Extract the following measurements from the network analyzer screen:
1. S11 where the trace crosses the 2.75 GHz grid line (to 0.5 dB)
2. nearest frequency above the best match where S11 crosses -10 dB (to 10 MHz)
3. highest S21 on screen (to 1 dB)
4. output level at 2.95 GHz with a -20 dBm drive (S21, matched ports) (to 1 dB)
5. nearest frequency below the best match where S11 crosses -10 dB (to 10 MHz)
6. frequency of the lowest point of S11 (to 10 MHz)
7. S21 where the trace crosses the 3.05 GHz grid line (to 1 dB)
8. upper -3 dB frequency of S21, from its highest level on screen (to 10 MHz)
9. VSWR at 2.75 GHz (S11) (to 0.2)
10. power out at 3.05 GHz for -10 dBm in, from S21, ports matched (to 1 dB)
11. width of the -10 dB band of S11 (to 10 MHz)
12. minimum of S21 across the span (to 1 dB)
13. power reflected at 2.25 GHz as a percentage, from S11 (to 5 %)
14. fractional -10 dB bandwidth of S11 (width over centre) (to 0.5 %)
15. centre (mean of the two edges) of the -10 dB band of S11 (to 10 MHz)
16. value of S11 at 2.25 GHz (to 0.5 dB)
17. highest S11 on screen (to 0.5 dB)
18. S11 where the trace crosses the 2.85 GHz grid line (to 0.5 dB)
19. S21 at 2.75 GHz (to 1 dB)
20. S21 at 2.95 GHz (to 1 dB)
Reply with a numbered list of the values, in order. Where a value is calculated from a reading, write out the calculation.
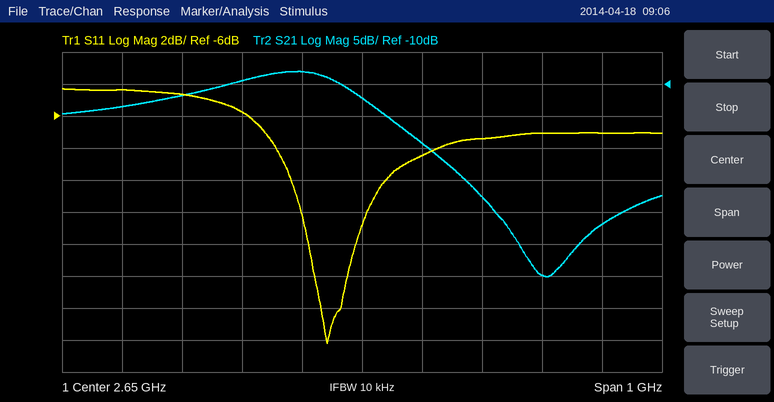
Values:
1. -8.5 dB
2. 2.69 GHz
3. -8 dB
4. -20 dBm + (-40 dB) = -60 dBm
5. 2.53 GHz
6. 2.59 GHz
7. -32 dB
8. 2.63 GHz
9. |Γ| = 10^(-8.5/20) = 0.3758; VSWR = (1 + 0.3758)/(1 − 0.3758) ≈ 2.2
10. -10 dBm + (-32 dB) = -42 dBm
11. 2.69 GHz − 2.53 GHz = 160 MHz
12. -40 dB
13. 10^(-4.5/10) ≈ 35 %
14. 160 MHz / 2.61 GHz ≈ 6.13 %, so 6.0 % to the nearest 0.5 %
15. 2.61 GHz
16. -4.5 dB
17. -4.5 dB
18. -7.5 dB
19. -19 dB
20. -40 dB
